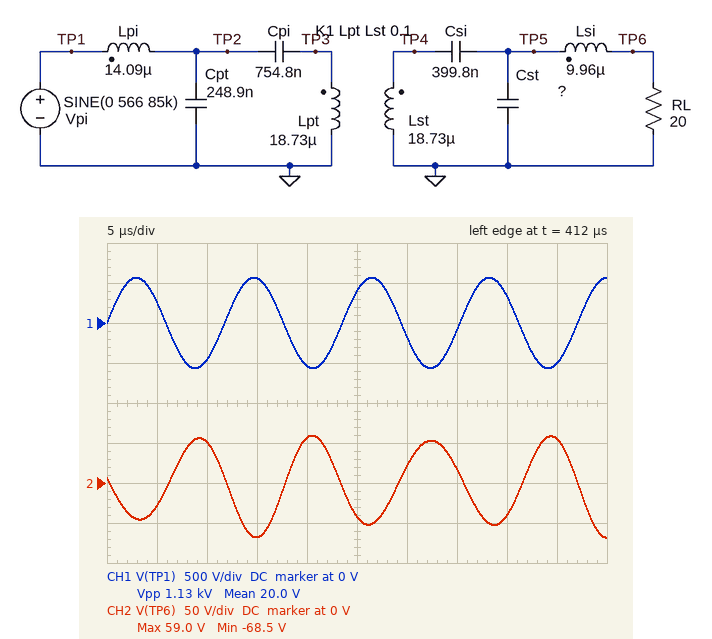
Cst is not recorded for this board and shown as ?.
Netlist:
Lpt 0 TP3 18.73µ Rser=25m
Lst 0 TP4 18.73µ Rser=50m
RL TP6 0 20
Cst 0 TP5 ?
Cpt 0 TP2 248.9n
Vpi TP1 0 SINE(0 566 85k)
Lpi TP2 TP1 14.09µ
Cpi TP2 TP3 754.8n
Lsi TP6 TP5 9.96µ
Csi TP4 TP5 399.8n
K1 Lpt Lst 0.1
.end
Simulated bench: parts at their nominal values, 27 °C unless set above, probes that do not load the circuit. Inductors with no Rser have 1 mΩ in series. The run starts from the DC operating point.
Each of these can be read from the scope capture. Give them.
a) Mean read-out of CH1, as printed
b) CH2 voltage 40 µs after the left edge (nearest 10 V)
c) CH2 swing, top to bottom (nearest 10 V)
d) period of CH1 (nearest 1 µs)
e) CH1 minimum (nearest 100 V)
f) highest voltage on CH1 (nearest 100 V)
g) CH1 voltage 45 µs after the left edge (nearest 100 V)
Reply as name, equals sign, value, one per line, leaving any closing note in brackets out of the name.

Mean read-out of CH1, as printed = 20.0 V
CH2 voltage 40 µs after the left edge = -40 V
CH2 swing, top to bottom = 130 V
period of CH1 = 12 µs
CH1 minimum = -600 V
highest voltage on CH1 = 600 V
CH1 voltage 45 µs after the left edge = -500 V
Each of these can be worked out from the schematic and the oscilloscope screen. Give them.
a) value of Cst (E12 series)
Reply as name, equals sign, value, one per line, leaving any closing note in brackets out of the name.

value of Cst = 820 nF
